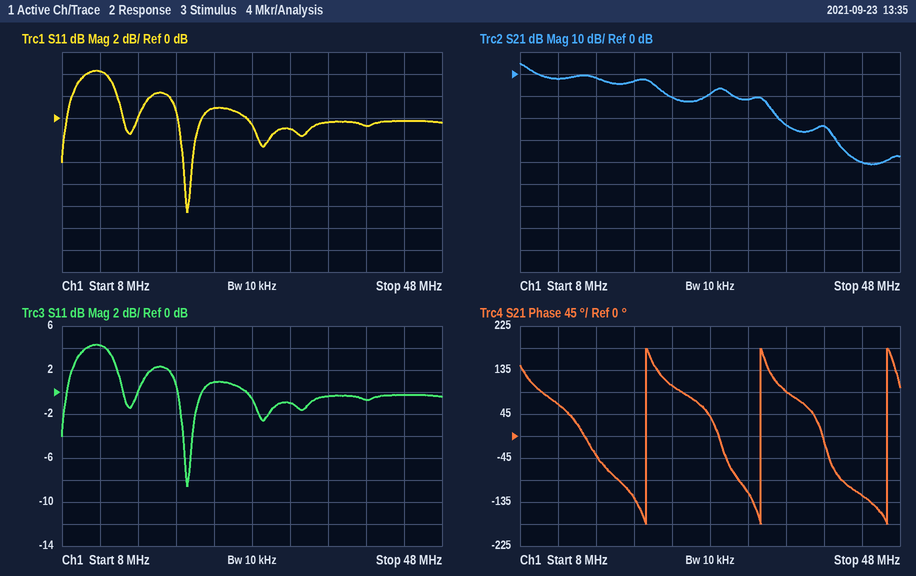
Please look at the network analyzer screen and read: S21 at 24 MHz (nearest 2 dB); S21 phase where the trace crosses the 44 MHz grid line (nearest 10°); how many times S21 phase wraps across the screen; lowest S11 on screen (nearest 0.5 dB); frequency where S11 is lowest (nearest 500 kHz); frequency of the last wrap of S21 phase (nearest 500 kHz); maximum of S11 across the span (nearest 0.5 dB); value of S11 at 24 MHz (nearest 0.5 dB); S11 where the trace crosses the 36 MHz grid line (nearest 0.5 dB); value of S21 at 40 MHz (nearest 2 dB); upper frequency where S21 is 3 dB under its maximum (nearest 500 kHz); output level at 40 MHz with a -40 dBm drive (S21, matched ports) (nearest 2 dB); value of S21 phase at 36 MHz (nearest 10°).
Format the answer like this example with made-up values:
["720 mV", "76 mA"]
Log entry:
["-10 dB", "-120°", "3", "-8.5 dB", "21.0 MHz", "46.5 MHz", "4.5 dB", "1.0 dB", "-0.5 dB", "-24 dB", "9.0 MHz", "-64 dBm", "90°"]
